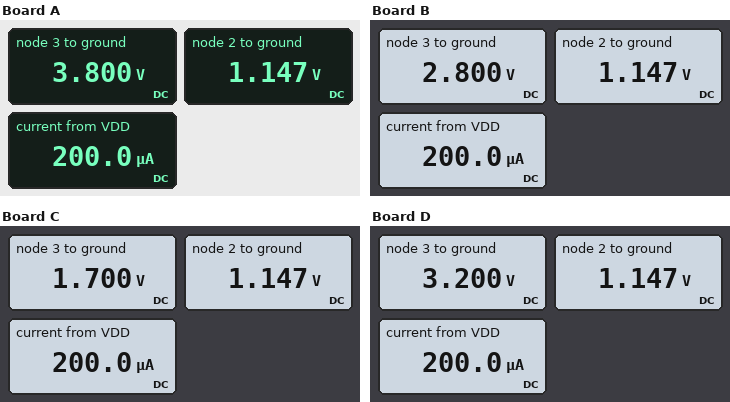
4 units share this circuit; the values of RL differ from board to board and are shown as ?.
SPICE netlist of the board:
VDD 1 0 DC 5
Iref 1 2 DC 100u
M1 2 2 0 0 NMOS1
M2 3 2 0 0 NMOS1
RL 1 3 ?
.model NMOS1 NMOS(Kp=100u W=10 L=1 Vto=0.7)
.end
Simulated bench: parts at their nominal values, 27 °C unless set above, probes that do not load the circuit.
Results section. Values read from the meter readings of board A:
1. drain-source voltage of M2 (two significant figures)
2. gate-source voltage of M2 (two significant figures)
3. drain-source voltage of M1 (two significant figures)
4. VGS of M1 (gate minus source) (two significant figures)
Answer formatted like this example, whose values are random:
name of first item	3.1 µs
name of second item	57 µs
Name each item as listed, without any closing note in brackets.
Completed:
drain-source voltage of M2	3.8 V
gate-source voltage of M2	1.1 V
drain-source voltage of M1	1.1 V
VGS of M1 (gate minus source)	1.1 V
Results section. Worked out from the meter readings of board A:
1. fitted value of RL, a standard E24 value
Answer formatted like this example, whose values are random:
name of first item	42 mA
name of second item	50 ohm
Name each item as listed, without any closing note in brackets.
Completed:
fitted value of RL, a standard E24 value	12 kΩ
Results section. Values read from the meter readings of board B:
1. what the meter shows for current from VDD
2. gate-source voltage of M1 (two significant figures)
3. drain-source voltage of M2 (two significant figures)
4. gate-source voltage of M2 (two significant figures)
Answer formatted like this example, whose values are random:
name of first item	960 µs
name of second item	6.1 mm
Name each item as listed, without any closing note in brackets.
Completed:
what the meter shows for current from VDD	200.0 µA
gate-source voltage of M1	1.1 V
drain-source voltage of M2	2.8 V
gate-source voltage of M2	1.1 V
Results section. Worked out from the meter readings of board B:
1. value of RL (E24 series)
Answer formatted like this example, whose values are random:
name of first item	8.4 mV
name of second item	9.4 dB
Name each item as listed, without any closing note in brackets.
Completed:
value of RL	22 kΩ
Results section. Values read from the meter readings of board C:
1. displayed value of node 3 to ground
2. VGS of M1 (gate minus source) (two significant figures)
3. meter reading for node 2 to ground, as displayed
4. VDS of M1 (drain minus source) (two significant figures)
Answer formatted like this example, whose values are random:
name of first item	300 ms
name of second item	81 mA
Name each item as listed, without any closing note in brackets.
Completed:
displayed value of node 3 to ground	1.700 V
VGS of M1 (gate minus source)	1.1 V
meter reading for node 2 to ground, as displayed	1.147 V
VDS of M1 (drain minus source)	1.1 V
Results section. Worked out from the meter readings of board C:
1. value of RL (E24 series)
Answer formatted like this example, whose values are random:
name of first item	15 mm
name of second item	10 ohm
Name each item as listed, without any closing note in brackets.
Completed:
value of RL	33 kΩ
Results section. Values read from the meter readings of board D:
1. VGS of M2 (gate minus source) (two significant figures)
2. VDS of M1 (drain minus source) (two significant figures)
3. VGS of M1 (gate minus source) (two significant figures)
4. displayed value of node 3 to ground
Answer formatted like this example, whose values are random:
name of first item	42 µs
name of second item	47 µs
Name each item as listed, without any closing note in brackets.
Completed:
VGS of M2 (gate minus source)	1.1 V
VDS of M1 (drain minus source)	1.1 V
VGS of M1 (gate minus source)	1.1 V
displayed value of node 3 to ground	3.200 V
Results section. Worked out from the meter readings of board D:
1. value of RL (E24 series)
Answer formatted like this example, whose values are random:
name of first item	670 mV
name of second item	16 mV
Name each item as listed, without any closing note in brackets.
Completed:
value of RL	18 kΩ
